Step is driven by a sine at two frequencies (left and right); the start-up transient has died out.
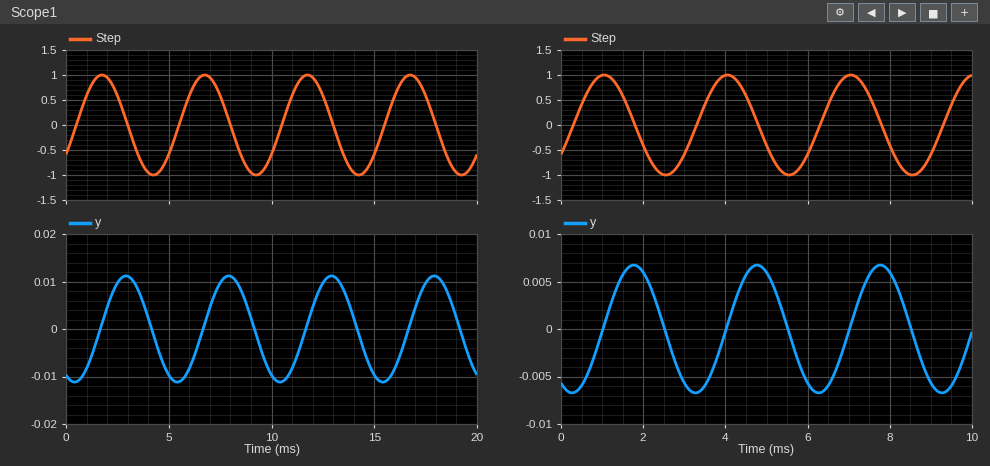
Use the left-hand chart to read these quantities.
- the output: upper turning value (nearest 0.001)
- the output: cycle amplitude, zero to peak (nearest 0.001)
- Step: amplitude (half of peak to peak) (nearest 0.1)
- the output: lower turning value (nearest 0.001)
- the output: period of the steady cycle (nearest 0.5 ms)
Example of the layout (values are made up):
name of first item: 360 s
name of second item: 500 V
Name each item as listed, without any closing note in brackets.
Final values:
the output: upper turning value: 0.011
the output: cycle amplitude, zero to peak: 0.011
Step: amplitude (half of peak to peak): 1.0
the output: lower turning value: -0.011
the output: period of the steady cycle: 5.0 ms
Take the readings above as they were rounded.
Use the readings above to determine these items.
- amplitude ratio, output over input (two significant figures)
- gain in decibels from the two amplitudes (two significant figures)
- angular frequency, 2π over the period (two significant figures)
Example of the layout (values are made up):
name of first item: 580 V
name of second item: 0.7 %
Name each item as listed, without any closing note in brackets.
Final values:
amplitude ratio, output over input: 0.011
gain in decibels from the two amplitudes: -39 dB
angular frequency, 2π over the period: 1.3 rad/ms
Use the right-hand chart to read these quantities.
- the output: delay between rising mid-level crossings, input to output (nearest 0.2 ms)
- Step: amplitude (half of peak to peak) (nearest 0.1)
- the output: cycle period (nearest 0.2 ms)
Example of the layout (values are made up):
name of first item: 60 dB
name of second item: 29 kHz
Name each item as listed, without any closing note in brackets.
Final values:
the output: delay between rising mid-level crossings, input to output: 0.8 ms
Step: amplitude (half of peak to peak): 1.0
the output: cycle period: 3.0 ms
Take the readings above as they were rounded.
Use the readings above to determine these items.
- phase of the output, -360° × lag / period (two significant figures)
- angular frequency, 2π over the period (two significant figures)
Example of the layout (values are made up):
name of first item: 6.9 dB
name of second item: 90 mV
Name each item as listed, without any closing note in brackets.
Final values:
phase of the output, -360° × lag / period: -96°
angular frequency, 2π over the period: 2.1 rad/ms
